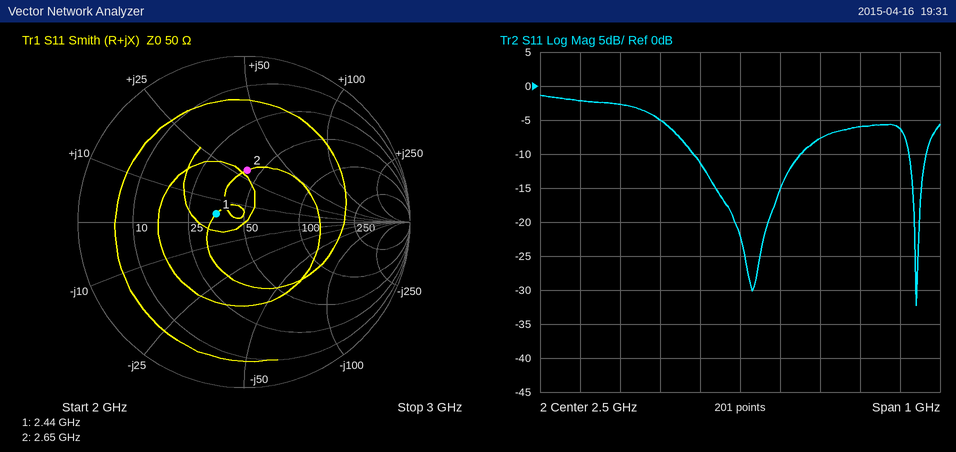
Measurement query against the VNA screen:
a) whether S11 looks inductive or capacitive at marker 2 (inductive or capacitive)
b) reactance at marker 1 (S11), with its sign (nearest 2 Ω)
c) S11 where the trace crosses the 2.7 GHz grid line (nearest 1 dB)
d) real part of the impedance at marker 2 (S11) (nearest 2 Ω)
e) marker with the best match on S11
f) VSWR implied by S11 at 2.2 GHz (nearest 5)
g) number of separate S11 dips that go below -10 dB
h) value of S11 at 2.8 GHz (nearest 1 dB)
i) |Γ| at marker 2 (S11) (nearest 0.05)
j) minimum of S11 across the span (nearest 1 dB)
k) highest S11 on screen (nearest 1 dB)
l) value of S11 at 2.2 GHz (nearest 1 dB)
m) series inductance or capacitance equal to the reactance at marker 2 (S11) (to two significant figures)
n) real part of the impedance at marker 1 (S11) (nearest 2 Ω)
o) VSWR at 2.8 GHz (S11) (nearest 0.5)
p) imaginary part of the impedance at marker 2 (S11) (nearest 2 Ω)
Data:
inductive
+4 Ω
-8 dB
42 Ω
marker 1
5
2
-6 dB
0.30
-32 dB
-1 dB
-3 dB
1.8 nH
36 Ω
3.0
+30 Ω
